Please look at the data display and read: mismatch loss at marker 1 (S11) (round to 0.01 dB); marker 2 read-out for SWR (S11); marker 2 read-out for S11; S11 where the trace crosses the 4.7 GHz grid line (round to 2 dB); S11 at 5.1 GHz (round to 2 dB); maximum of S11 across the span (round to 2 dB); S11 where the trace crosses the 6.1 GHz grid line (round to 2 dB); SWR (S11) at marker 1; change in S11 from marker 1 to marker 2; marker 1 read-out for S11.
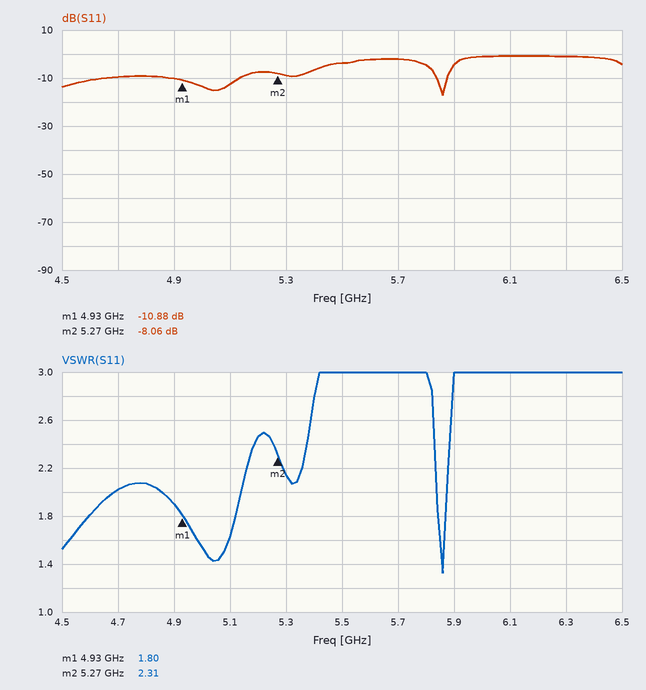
0.37 dB
2.31
-8.06 dB
-10 dB
-12 dB
0 dB
0 dB
1.80
2.82 dB
-10.88 dB
